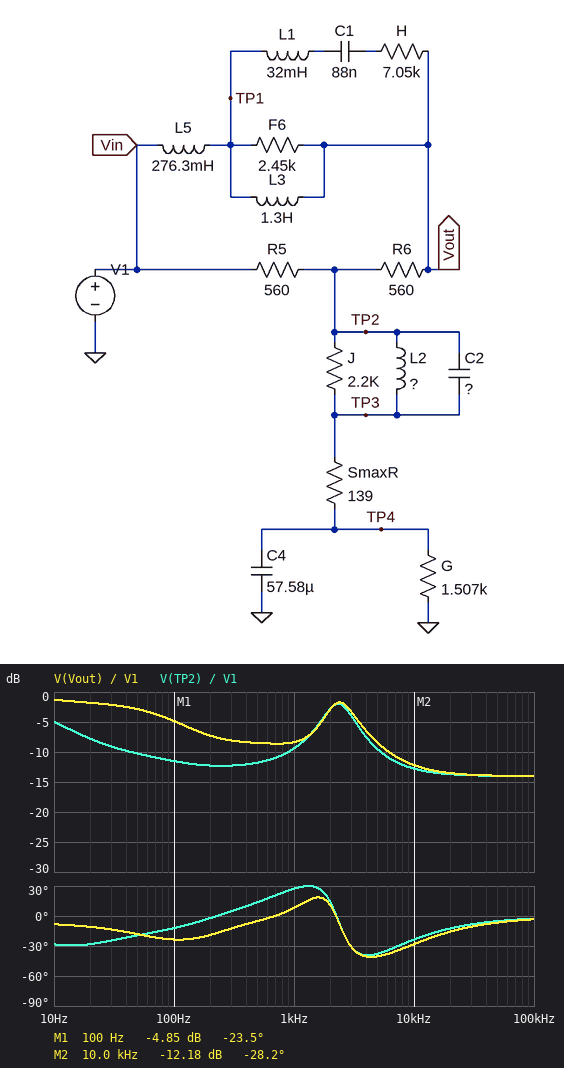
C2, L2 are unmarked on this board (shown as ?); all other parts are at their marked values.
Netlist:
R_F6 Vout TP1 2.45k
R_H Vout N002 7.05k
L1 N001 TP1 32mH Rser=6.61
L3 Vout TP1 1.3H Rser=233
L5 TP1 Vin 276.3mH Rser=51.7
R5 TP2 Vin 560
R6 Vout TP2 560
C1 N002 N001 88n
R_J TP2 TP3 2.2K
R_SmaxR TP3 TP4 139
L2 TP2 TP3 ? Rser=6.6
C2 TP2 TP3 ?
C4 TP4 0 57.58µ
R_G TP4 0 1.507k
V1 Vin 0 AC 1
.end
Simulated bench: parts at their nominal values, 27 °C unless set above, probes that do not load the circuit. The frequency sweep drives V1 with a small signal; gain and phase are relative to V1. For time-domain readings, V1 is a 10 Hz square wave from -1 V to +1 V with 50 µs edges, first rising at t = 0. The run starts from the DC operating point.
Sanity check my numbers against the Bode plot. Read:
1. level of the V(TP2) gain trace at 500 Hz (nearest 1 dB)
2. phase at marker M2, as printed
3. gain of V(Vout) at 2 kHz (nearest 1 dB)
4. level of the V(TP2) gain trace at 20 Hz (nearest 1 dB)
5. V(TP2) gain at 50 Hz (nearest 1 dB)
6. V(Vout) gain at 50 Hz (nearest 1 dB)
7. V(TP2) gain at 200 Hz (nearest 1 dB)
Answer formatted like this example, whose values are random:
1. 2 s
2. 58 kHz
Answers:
1. -12 dB
2. -28.2 deg
3. -3 dB
4. -8 dB
5. -10 dB
6. -3 dB
7. -12 dB
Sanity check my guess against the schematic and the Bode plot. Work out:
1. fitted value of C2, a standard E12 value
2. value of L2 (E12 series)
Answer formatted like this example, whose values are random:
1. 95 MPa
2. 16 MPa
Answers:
1. 220 nF
2. 22 mH
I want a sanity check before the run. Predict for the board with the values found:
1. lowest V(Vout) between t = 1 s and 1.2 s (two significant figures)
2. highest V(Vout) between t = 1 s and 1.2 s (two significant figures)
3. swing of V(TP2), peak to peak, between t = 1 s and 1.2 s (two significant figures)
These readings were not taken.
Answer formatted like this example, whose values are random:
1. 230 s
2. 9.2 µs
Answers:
1. -920 mV
2. 920 mV
3. 1.5 V
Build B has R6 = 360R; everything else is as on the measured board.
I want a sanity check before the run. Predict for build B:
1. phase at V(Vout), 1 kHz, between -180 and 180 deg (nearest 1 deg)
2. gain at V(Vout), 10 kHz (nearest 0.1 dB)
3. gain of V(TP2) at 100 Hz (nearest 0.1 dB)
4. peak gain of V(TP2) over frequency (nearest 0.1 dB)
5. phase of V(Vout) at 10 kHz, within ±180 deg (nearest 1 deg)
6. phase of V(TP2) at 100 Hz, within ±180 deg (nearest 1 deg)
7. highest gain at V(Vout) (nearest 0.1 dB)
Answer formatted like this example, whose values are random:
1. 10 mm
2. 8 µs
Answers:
1. 13 deg
2. -12.4 dB
3. -11.4 dB
4. -1.4 dB
5. -27 deg
6. -14 deg
7. -0.6 dB
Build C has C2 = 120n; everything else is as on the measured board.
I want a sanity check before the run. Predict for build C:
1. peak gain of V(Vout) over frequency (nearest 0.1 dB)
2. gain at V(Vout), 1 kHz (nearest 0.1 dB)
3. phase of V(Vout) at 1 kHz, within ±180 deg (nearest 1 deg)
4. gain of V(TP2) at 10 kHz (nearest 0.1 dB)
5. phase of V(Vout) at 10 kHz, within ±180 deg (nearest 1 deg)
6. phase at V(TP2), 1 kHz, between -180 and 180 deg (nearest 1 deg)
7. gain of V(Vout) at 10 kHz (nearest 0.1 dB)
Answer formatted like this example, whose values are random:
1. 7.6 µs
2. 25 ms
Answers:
1. -0.5 dB
2. -8.6 dB
3. 6 deg
4. -10.7 dB
5. -37 deg
6. 26 deg
7. -10.1 dB
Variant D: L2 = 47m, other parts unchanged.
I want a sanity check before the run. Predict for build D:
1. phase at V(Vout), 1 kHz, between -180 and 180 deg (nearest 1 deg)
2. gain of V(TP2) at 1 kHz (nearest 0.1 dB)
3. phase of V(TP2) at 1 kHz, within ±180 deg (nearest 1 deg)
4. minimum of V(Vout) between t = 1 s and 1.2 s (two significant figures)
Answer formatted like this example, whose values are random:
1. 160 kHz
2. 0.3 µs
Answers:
1. 17 deg
2. -4.6 dB
3. 26 deg
4. -920 mV
